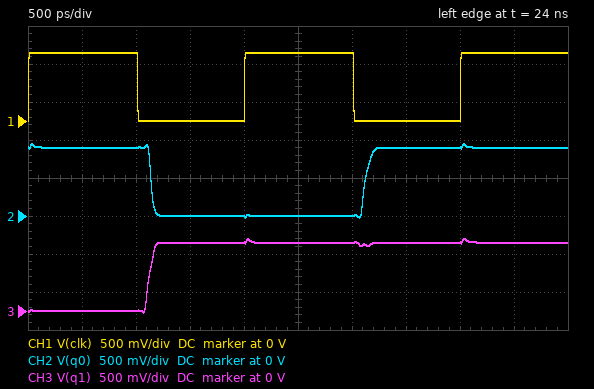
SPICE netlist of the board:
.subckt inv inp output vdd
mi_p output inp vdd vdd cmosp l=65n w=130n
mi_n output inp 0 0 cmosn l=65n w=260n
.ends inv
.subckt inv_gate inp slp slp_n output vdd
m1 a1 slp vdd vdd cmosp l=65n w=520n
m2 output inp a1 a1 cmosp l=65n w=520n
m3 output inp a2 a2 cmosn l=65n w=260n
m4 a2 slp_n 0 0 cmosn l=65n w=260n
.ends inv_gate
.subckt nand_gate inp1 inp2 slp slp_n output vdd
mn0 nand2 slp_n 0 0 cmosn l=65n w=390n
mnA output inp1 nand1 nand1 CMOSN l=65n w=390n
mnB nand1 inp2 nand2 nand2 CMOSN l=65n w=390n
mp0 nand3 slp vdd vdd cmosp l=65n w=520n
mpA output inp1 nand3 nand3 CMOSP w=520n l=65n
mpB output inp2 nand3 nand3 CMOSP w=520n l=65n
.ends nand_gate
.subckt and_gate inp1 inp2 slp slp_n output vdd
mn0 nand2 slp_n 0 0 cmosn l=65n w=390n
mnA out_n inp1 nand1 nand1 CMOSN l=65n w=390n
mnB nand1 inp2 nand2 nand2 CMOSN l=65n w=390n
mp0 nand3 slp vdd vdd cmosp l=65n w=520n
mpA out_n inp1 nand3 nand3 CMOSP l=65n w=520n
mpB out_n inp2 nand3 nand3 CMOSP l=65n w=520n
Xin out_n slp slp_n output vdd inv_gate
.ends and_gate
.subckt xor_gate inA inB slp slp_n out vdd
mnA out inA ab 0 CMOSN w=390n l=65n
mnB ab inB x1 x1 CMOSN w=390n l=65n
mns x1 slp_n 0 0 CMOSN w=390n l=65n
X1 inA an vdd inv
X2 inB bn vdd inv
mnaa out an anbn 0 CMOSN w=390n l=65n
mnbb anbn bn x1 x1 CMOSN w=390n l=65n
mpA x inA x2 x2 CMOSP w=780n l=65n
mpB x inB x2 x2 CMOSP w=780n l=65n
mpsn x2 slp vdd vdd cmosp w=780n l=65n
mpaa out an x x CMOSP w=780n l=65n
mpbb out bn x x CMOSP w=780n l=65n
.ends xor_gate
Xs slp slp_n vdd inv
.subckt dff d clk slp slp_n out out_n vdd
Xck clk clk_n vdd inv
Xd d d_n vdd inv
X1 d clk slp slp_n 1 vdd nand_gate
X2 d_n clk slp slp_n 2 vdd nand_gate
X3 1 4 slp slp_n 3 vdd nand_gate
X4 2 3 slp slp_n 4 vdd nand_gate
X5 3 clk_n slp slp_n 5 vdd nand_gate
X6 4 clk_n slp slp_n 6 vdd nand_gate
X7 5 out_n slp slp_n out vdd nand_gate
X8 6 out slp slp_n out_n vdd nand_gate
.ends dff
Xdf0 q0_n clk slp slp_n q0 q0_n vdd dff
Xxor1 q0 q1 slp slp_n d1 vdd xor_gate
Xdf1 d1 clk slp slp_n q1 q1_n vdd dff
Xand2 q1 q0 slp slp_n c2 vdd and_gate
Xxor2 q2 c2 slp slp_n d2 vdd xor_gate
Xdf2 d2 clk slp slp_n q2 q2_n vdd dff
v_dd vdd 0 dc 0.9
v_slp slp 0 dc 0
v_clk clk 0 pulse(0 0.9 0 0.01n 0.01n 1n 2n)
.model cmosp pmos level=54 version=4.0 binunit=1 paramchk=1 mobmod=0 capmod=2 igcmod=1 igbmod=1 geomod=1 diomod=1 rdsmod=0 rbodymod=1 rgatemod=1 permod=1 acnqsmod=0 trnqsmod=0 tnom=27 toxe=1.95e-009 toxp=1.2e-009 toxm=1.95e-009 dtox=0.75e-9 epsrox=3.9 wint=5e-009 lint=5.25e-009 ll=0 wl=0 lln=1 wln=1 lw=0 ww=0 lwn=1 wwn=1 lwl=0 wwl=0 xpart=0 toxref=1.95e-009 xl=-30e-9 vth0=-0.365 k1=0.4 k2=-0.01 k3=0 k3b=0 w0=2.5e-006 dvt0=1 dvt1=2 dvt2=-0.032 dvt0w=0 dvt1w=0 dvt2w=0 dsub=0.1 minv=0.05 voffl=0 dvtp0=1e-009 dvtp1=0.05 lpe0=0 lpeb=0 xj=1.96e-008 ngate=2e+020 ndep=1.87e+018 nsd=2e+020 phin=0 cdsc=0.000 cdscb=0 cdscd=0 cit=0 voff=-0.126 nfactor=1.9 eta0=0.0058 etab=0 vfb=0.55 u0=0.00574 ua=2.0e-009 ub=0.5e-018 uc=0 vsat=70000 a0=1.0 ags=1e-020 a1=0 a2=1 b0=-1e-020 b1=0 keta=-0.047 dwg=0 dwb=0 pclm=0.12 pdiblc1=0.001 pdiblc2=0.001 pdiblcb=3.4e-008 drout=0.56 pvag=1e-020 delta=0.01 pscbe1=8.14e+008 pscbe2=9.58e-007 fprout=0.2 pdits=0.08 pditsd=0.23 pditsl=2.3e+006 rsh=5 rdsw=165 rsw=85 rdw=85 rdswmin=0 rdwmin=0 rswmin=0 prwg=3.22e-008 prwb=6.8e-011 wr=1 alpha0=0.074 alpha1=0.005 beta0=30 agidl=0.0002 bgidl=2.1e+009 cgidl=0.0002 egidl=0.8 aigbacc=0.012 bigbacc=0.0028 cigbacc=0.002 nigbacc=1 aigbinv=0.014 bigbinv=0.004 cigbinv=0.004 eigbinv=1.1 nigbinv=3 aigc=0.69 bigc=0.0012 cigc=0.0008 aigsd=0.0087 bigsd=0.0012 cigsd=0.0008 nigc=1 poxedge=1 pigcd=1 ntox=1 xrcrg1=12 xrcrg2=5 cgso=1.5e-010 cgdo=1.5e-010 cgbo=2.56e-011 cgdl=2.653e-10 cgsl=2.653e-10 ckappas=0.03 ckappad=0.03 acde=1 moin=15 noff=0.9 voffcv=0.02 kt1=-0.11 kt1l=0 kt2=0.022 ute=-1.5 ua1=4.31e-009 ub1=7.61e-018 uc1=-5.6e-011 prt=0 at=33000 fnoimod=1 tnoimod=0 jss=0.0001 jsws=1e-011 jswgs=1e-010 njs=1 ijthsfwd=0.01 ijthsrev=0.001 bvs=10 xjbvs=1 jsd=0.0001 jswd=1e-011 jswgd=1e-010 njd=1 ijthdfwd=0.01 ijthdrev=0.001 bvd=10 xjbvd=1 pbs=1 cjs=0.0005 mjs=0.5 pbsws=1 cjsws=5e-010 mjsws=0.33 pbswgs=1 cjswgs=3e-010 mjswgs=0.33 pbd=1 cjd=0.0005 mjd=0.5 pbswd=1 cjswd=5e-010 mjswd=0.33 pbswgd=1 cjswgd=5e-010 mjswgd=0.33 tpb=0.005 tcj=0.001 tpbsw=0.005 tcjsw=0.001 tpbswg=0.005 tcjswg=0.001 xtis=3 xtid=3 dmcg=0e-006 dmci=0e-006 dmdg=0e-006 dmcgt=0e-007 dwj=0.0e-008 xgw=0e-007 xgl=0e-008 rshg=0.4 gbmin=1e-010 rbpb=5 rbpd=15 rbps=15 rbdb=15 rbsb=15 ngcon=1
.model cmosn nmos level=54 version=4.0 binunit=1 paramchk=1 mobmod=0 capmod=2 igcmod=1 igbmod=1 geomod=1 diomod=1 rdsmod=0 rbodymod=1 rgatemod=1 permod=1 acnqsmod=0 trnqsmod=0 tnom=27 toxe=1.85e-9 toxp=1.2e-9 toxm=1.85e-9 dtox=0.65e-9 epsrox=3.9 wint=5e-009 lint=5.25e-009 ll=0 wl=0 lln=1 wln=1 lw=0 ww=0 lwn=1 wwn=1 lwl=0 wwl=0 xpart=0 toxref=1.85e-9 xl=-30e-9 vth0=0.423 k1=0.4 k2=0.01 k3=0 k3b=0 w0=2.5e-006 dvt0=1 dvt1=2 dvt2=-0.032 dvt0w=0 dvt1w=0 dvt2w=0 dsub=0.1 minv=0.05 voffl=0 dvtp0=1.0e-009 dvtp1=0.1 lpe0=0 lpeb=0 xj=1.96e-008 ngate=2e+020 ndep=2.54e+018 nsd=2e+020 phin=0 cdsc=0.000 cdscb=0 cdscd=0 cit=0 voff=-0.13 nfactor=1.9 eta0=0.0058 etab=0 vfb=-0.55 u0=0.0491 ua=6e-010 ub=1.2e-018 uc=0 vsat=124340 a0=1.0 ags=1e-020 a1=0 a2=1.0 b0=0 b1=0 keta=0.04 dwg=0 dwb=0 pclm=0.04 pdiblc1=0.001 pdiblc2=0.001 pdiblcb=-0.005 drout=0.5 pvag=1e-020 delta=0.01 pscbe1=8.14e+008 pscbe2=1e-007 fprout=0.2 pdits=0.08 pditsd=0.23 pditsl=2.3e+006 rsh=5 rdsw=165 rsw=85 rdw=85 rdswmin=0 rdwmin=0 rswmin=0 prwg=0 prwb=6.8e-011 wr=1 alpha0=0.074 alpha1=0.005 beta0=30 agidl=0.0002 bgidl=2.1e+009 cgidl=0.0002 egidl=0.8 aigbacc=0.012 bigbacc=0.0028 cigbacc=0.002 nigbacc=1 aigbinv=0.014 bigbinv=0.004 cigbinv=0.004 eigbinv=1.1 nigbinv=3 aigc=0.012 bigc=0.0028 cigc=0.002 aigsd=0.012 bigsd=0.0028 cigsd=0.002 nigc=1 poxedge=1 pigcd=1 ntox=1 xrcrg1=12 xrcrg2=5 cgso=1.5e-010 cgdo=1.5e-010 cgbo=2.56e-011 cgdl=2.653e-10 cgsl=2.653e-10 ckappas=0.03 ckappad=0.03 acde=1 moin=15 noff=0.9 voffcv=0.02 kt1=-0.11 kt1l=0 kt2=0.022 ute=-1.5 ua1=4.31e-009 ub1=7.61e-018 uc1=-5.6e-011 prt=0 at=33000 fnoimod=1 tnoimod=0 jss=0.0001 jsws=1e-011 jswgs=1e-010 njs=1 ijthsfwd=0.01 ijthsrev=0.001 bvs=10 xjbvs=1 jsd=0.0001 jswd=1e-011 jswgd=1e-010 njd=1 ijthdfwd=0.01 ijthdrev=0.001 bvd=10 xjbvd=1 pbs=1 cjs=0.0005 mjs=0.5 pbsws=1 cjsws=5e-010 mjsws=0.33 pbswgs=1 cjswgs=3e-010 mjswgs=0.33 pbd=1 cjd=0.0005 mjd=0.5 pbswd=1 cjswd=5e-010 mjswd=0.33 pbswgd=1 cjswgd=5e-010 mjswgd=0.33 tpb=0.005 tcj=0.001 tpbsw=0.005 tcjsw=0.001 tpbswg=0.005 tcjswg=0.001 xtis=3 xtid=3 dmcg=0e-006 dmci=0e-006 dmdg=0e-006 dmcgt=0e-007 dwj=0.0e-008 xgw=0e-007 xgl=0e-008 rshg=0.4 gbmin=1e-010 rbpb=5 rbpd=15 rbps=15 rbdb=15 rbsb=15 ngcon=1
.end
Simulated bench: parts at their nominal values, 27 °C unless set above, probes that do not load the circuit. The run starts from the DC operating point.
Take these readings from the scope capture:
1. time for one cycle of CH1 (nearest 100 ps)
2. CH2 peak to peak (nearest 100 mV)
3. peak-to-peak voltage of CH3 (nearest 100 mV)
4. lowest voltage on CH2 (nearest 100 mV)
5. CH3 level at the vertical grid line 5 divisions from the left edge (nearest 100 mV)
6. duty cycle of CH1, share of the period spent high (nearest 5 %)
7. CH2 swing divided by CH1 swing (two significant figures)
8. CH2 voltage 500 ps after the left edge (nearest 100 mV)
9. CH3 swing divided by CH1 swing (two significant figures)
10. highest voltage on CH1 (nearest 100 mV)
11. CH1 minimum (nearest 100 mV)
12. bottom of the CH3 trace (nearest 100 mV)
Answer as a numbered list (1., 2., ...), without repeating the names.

1. 2.0 ns
2. 1.0 V
3. 1.0 V
4. 0 V
5. 900 mV
6. 50 %
7. 1.1
8. 900 mV
9. 1.1
10. 900 mV
11. 0 V
12. 0 V
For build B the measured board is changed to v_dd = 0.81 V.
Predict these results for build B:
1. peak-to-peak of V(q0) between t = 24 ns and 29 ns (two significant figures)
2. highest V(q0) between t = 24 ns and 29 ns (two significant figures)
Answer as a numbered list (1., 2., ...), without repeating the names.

1. 880 mV
2. 850 mV
